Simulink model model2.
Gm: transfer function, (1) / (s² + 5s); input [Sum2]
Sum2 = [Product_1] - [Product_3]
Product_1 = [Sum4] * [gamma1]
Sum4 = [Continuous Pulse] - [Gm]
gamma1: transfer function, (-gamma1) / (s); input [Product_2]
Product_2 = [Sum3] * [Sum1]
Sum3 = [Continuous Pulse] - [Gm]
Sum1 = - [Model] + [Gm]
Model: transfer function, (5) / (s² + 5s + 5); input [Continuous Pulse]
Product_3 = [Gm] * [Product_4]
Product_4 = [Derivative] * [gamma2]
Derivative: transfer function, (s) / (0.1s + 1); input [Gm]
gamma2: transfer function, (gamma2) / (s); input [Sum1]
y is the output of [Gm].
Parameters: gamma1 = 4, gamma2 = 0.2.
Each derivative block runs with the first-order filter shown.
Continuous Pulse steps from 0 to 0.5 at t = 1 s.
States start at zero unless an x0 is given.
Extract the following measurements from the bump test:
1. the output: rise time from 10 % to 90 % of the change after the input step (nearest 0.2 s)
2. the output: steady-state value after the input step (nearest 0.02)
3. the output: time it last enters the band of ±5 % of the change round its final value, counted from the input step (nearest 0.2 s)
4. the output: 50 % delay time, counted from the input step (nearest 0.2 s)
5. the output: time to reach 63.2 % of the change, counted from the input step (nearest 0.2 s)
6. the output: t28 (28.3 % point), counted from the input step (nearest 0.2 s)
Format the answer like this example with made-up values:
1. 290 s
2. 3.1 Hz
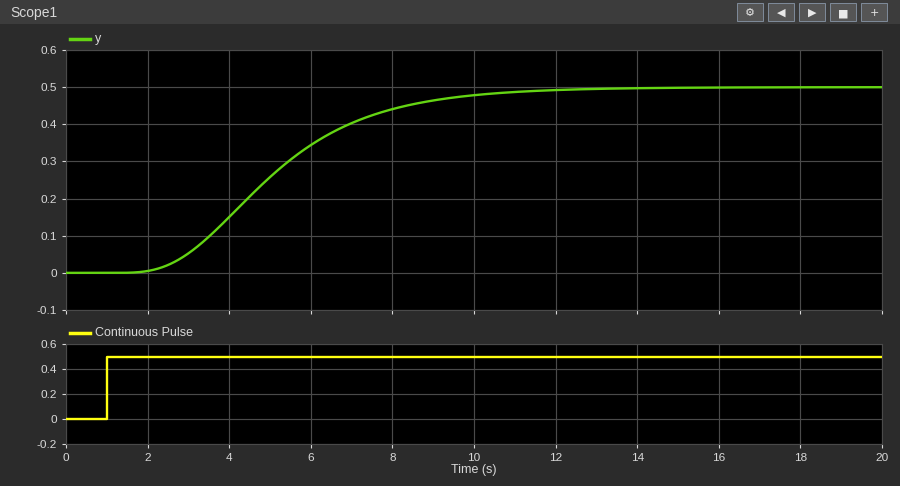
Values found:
1. 5.4 s
2. 0.50
3. 8.8 s
4. 4.0 s
5. 4.6 s
6. 3.0 s
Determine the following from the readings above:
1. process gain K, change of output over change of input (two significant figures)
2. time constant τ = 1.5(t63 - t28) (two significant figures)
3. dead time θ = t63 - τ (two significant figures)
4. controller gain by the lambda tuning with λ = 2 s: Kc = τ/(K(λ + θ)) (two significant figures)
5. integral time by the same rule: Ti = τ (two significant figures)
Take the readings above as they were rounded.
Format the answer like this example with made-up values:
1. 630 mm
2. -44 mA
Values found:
1. 1.0
2. 2.4 s
3. 2.2 s
4. 0.57
5. 2.4 s
